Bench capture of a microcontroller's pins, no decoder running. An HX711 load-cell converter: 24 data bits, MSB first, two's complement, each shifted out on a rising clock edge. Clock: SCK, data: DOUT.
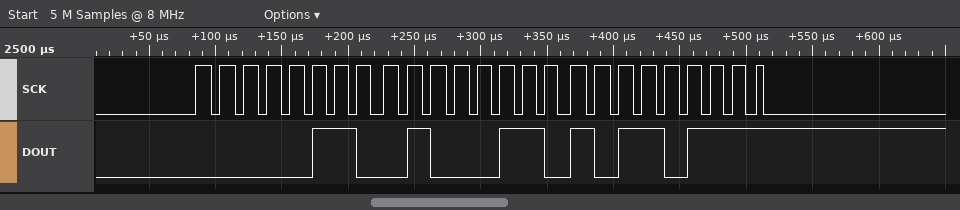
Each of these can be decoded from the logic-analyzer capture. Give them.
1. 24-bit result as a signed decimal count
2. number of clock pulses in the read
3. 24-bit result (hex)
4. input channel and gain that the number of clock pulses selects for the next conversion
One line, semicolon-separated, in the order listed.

411319; 25; 0x0646B7; channel A, gain 128
